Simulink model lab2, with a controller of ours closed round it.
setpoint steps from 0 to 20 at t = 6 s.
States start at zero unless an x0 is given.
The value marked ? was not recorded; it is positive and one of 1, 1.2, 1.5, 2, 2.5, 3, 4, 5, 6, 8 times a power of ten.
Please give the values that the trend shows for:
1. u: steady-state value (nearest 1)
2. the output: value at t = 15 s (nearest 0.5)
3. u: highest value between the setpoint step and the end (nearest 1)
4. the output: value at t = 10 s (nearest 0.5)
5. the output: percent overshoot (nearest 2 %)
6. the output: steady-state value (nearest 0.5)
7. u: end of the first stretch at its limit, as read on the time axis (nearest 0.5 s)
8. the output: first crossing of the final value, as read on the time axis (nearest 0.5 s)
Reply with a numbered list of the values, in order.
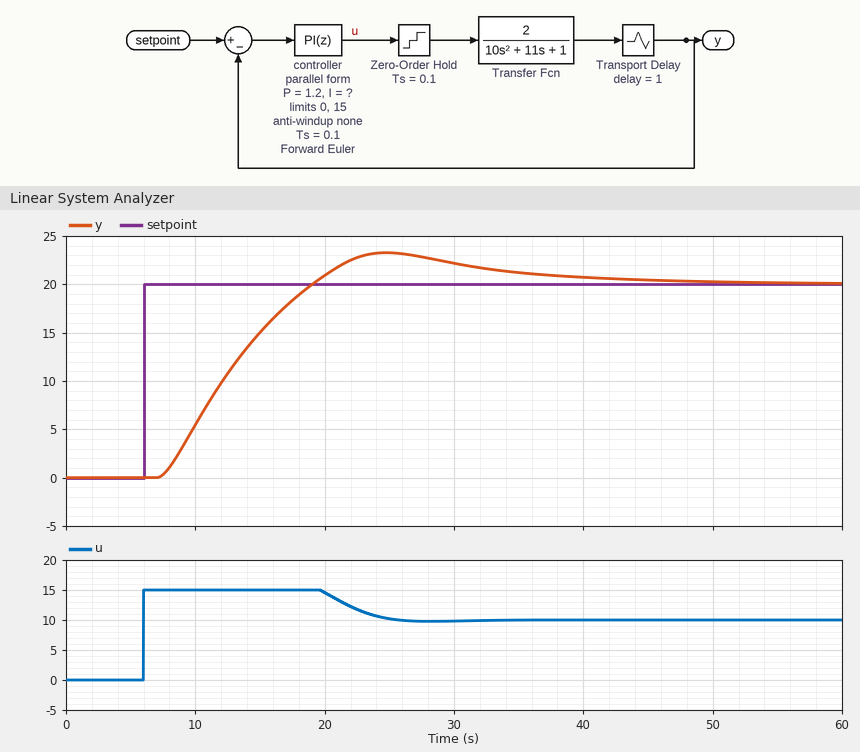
1. 10
2. 15.0
3. 15
4. 5.5
5. 16 %
6. 20.0
7. 20.0 s
8. 19.0 s
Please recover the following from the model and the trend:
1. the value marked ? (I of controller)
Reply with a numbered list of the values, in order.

1. 0.12
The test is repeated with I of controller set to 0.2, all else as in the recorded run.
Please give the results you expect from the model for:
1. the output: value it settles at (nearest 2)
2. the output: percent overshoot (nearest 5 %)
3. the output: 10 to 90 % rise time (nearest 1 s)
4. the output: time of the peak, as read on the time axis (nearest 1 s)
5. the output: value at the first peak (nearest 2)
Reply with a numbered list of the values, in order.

1. 20
2. 30 %
3. 9 s
4. 30 s
5. 26
